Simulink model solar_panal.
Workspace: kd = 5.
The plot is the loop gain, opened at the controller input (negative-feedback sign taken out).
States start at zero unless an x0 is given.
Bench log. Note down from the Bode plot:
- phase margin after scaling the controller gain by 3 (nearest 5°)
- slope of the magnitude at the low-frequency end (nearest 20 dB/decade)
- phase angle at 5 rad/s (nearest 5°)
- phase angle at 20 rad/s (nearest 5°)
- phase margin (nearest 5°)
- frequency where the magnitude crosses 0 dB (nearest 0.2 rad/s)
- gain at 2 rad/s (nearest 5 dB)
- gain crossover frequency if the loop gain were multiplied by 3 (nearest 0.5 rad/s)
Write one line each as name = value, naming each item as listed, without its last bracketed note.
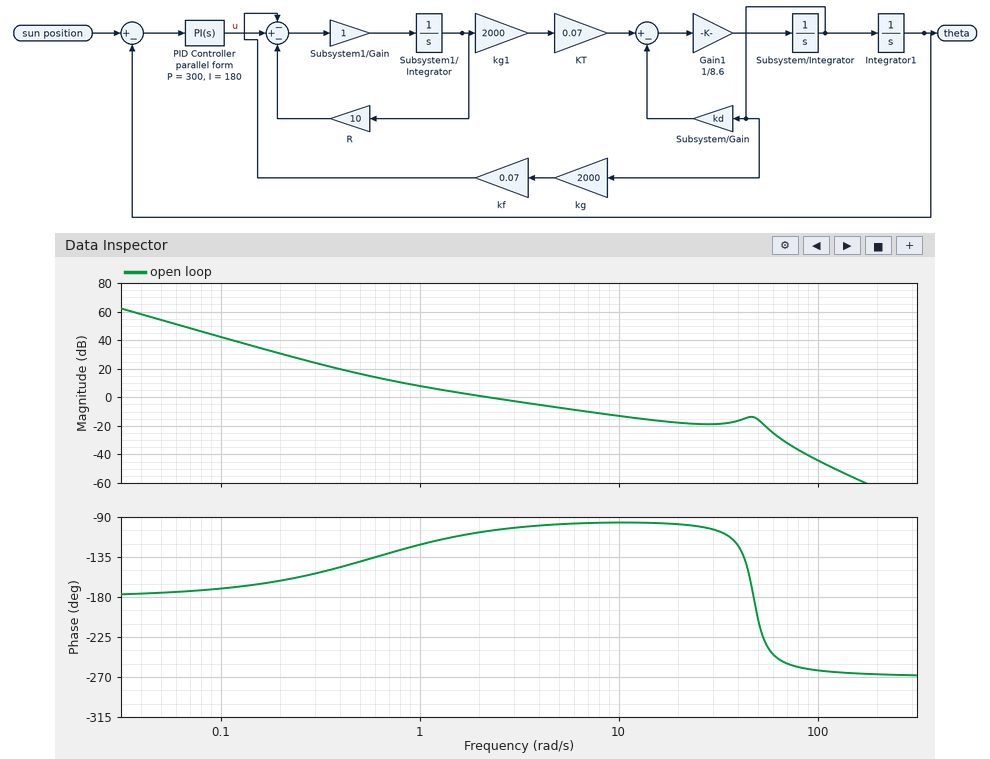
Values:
phase margin after scaling the controller gain by 3 = 85°
slope of the magnitude at the low-frequency end = -40 dB/decade
phase angle at 5 rad/s = -100°
phase angle at 20 rad/s = -100°
phase margin = 75°
frequency where the magnitude crosses 0 dB = 2.2 rad/s
gain at 2 rad/s = 0 dB
gain crossover frequency if the loop gain were multiplied by 3 = 6.5 rad/s
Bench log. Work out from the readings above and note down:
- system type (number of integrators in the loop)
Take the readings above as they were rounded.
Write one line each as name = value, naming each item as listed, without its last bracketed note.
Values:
system type = 2
